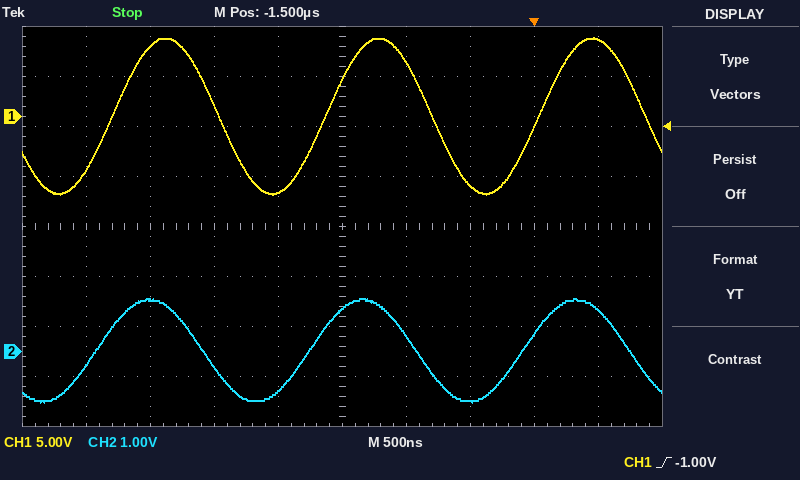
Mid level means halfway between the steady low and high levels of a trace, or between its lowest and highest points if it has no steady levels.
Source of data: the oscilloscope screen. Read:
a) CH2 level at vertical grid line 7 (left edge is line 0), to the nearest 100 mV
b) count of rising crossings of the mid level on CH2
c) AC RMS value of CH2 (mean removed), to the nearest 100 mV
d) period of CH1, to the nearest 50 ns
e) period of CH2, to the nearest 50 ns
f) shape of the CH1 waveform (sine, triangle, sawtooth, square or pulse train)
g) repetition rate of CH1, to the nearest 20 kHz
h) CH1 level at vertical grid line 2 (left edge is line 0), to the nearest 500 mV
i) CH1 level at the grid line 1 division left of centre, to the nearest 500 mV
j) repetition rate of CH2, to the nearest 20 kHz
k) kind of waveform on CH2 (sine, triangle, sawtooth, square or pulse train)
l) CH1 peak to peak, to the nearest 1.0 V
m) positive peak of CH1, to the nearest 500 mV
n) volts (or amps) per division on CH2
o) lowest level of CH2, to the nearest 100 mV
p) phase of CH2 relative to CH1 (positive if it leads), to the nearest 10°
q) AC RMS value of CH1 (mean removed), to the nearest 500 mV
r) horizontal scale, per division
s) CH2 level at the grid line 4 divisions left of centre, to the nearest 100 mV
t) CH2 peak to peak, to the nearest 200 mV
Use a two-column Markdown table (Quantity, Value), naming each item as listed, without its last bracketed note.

| Quantity | Value |
|---|---|
| CH2 level at vertical grid line 7 (left edge is line 0), to the nearest 100 mV | -1.0 V |
| count of rising crossings of the mid level on CH2 | 3 |
| AC RMS value of CH2 (mean removed), to the nearest 100 mV | 700 mV |
| period of CH1, to the nearest 50 ns | 1.65 µs |
| period of CH2, to the nearest 50 ns | 1.65 µs |
| shape of the CH1 waveform | sine |
| repetition rate of CH1, to the nearest 20 kHz | 600 kHz |
| CH1 level at vertical grid line 2 (left edge is line 0), to the nearest 500 mV | 7.0 V |
| CH1 level at the grid line 1 division left of centre, to the nearest 500 mV | -7.5 V |
| repetition rate of CH2, to the nearest 20 kHz | 600 kHz |
| kind of waveform on CH2 | sine |
| CH1 peak to peak, to the nearest 1.0 V | 16.0 V |
| positive peak of CH1, to the nearest 500 mV | 8.0 V |
| volts (or amps) per division on CH2 | 1 V |
| lowest level of CH2, to the nearest 100 mV | -1.0 V |
| phase of CH2 relative to CH1 (positive if it leads), to the nearest 10° | +30° |
| AC RMS value of CH1 (mean removed), to the nearest 500 mV | 5.5 V |
| horizontal scale, per division | 500 ns |
| CH2 level at the grid line 4 divisions left of centre, to the nearest 100 mV | -300 mV |
| CH2 peak to peak, to the nearest 200 mV | 2.0 V |
